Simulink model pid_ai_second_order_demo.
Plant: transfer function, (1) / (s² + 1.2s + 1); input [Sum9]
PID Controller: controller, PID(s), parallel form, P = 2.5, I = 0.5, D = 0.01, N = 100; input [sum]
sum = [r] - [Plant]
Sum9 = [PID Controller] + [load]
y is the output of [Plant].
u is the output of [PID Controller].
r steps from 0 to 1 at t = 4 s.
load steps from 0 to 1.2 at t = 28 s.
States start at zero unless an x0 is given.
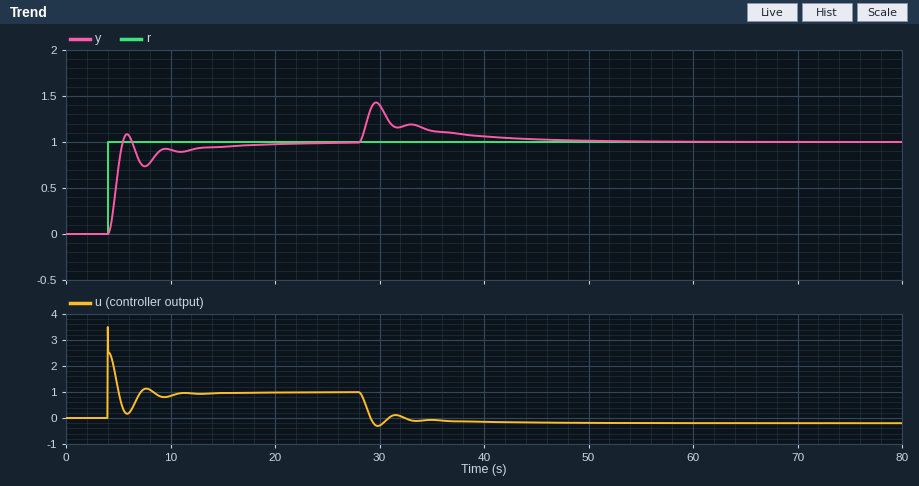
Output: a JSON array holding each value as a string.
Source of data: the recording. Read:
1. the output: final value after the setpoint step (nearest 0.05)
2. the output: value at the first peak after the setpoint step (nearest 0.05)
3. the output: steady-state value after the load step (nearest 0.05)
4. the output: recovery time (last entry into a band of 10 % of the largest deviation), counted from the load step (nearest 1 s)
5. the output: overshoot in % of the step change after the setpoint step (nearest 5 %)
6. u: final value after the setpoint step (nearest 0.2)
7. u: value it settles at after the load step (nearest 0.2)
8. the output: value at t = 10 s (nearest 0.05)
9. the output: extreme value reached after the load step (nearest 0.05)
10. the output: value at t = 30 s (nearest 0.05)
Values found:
["1.00", "1.10", "1.00", "14 s", "10 %", "1.0", "-0.2", "0.90", "1.45", "1.40"]
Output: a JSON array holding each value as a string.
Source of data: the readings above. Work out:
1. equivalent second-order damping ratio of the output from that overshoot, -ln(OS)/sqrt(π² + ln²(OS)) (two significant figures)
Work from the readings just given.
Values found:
["0.59"]
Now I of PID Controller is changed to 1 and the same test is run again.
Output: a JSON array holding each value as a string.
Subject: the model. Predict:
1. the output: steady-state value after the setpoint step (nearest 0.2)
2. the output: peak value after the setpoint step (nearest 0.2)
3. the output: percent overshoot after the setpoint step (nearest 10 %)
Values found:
["1.0", "1.2", "20 %"]
